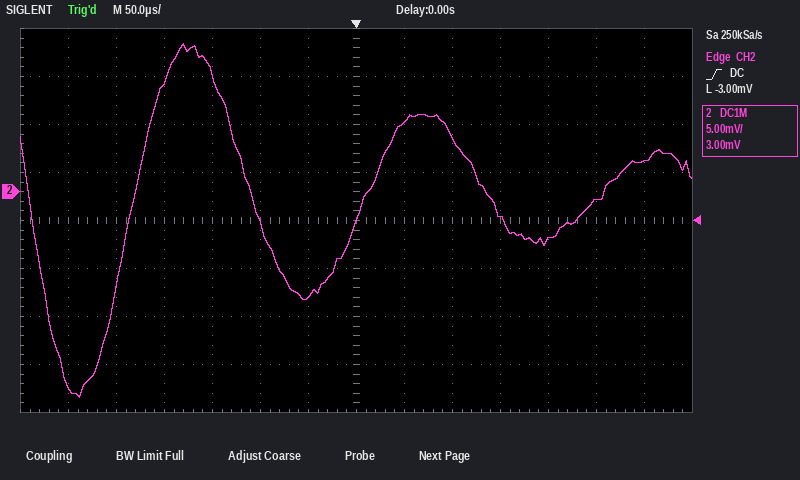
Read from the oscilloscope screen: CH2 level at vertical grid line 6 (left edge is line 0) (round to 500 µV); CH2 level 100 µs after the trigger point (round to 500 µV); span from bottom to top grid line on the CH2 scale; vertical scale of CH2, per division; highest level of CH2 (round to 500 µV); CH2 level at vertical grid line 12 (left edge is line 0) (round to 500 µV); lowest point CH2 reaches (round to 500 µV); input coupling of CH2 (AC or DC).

-11.0 mV
5.5 mV
40 mV
5 mV
15.5 mV
-1.0 mV
-21.5 mV
DC
